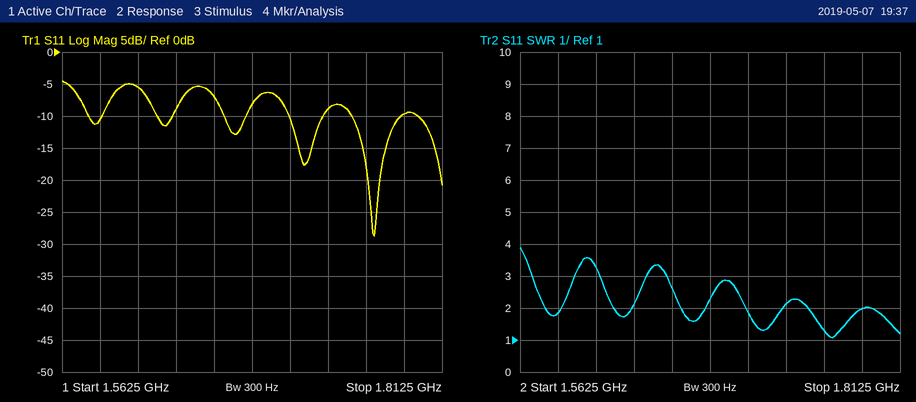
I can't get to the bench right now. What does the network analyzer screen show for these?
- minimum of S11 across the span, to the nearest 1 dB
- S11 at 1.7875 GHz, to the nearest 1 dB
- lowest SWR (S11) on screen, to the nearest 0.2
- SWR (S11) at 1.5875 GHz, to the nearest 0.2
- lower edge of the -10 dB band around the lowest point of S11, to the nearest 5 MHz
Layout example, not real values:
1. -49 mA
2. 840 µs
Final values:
1. -29 dB
2. -10 dB
3. 1.0
4. 1.8
5. 1.755 GHz
